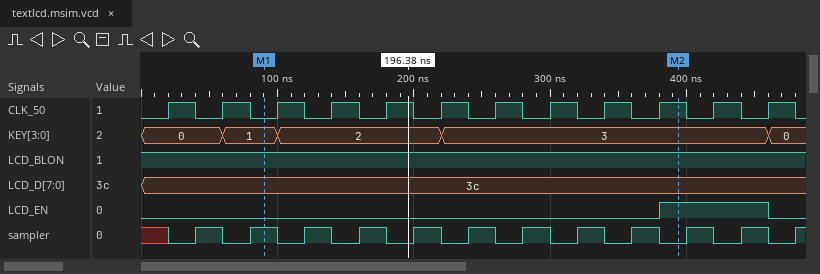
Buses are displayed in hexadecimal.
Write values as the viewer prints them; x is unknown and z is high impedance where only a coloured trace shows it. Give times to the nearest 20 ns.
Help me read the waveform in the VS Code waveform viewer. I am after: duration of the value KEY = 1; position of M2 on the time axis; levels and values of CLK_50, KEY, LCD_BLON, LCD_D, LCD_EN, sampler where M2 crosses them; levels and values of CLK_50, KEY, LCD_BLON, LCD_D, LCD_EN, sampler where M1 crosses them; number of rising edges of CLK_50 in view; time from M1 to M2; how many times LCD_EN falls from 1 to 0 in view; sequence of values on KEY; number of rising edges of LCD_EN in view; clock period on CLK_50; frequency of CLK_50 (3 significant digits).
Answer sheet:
40 ns
400 ns
CLK_50=1, KEY=3, LCD_BLON=1, LCD_D=3c, LCD_EN=1, sampler=0
CLK_50=0, KEY=1, LCD_BLON=1, LCD_D=3c, LCD_EN=0, sampler=1
12
300 ns
1
0, 1, 2, 3, 0
1
40 ns
25.0 MHz
